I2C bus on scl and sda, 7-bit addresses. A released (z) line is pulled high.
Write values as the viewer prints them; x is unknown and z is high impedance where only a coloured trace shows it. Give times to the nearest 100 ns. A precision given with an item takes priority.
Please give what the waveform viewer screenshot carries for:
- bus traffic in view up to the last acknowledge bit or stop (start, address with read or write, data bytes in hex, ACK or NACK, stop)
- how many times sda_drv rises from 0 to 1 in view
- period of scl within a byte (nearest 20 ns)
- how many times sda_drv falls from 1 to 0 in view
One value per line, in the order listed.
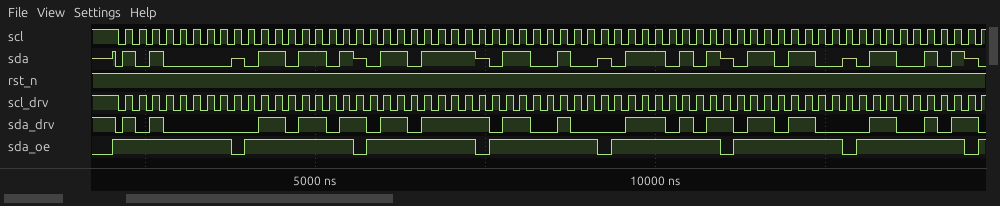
start, address 50 write NACK, 6D NACK, 6F NACK, 64 NACK, 75 NACK, 6C NACK, 65 NACK
17
200 ns
18
